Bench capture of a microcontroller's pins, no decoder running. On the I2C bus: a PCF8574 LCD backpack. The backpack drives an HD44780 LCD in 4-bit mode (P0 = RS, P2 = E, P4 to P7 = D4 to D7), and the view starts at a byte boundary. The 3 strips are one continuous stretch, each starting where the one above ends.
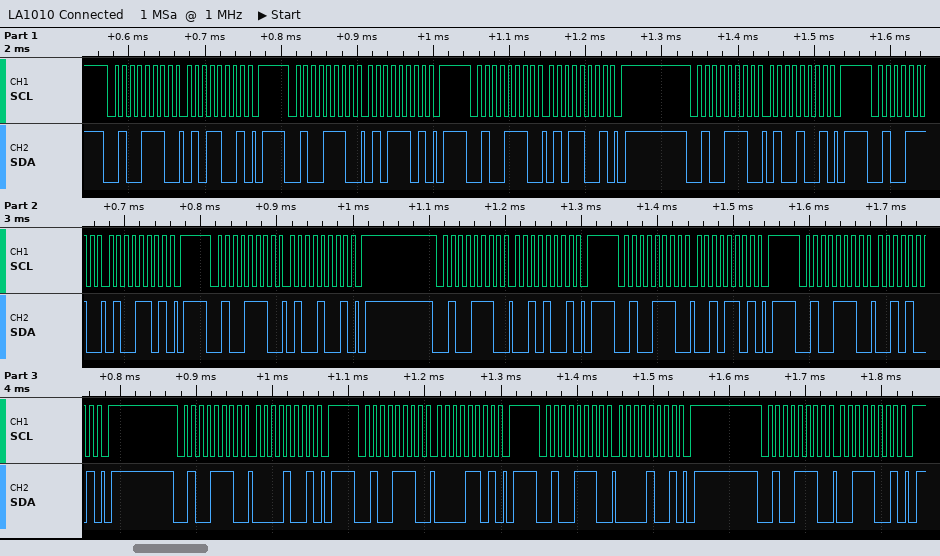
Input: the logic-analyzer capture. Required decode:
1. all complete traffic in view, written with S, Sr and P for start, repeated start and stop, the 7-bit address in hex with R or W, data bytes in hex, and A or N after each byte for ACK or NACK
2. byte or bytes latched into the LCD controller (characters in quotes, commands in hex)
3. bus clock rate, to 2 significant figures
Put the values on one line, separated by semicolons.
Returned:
S 27W A 59 A P S 27W A 5D A P S 27W A 59 A P S 27W A 49 A P S 27W A 4D A P S 27W A 49 A P S 27W A 29 A P S 27W A 2D A P S 27W A 29 A P S 27W A 09 A P S 27W A 0D A P S 27W A 09 A P S 27W A 39 A P; 'T' ' '; 100 kHz
